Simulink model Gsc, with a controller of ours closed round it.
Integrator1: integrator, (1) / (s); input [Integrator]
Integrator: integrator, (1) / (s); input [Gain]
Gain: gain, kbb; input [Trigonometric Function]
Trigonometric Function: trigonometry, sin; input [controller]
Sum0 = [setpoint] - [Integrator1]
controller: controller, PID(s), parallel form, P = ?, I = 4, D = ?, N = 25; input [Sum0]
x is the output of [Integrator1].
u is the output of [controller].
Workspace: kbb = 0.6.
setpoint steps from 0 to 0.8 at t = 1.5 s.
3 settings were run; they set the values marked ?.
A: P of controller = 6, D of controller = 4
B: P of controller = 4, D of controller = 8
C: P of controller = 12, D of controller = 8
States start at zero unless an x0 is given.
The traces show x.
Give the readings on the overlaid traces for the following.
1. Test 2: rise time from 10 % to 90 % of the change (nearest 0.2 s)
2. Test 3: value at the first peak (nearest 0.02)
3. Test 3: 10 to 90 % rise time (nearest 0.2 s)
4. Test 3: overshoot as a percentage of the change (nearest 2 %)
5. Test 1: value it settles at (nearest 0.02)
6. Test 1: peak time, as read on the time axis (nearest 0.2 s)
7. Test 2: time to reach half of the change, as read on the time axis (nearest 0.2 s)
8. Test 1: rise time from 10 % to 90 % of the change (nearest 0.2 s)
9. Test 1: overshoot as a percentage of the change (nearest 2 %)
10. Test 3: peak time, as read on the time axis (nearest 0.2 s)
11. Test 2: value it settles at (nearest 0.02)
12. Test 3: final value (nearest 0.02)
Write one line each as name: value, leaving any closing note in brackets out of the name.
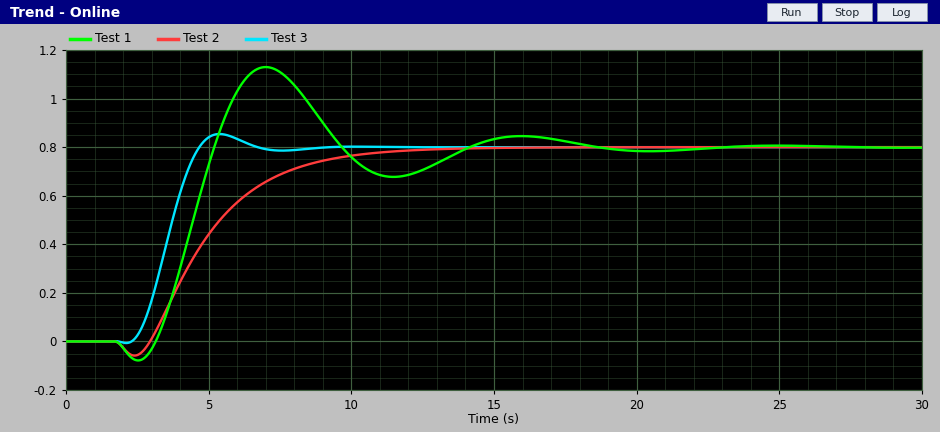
Test 2: rise time from 10 % to 90 % of the change: 5.0 s
Test 3: value at the first peak: 0.86
Test 3: 10 to 90 % rise time: 1.6 s
Test 3: overshoot as a percentage of the change: 6 %
Test 1: value it settles at: 0.80
Test 1: peak time, as read on the time axis: 7.0 s
Test 2: time to reach half of the change, as read on the time axis: 4.8 s
Test 1: rise time from 10 % to 90 % of the change: 1.6 s
Test 1: overshoot as a percentage of the change: 42 %
Test 3: peak time, as read on the time axis: 5.4 s
Test 2: value it settles at: 0.80
Test 3: final value: 0.80
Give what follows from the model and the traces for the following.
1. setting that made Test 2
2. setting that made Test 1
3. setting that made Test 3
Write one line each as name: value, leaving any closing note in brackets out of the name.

setting that made Test 2: C
setting that made Test 1: B
setting that made Test 3: A
